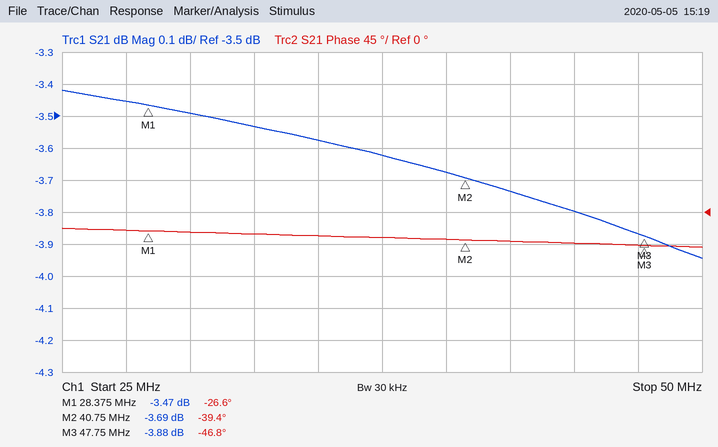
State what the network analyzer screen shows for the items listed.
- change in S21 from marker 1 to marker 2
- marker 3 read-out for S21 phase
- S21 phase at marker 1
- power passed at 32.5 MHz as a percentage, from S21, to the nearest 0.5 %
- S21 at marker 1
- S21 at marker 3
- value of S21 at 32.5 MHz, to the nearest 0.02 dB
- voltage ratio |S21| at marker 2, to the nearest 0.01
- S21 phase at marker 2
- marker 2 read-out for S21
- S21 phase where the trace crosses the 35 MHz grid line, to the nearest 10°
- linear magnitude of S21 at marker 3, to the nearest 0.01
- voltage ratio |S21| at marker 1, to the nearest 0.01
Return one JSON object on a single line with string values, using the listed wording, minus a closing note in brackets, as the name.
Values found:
{"change in S21 from marker 1 to marker 2": "-0.22 dB", "marker 3 read-out for S21 phase": "-46.8°", "S21 phase at marker 1": "-26.6°", "power passed at 32.5 MHz as a percentage, from S21, to the nearest 0.5 %": "44.5 %", "S21 at marker 1": "-3.47 dB", "S21 at marker 3": "-3.88 dB", "value of S21 at 32.5 MHz, to the nearest 0.02 dB": "-3.54 dB", "voltage ratio |S21| at marker 2, to the nearest 0.01": "0.65", "S21 phase at marker 2": "-39.4°", "marker 2 read-out for S21": "-3.69 dB", "S21 phase where the trace crosses the 35 MHz grid line, to the nearest 10°": "-30°", "linear magnitude of S21 at marker 3, to the nearest 0.01": "0.64", "voltage ratio |S21| at marker 1, to the nearest 0.01": "0.67"}
